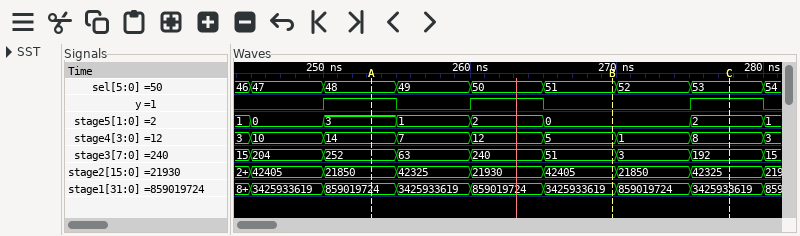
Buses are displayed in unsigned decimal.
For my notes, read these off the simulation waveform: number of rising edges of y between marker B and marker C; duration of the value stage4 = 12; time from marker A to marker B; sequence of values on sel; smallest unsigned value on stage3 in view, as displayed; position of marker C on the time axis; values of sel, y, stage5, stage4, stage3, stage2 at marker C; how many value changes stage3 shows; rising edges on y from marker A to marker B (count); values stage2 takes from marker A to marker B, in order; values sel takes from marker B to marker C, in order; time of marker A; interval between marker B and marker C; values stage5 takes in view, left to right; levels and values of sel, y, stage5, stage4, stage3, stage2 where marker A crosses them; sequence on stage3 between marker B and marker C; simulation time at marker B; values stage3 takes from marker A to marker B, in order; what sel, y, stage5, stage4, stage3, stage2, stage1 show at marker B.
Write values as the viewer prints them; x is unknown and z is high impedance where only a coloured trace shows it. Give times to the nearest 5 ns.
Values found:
1
5 ns
15 ns
46, 47, 48, 49, 50, 51, 52, 53, 54
3
280 ns
sel=53, y=1, stage5=2, stage4=8, stage3=192, stage2=42325
8
1
21850, 42325, 21930, 42405
51, 52, 53
255 ns
10 ns
1, 0, 3, 1, 2, 0, 2, 1
sel=48, y=1, stage5=3, stage4=14, stage3=252, stage2=21850
51, 3, 192
270 ns
252, 63, 240, 51
sel=51, y=0, stage5=0, stage4=5, stage3=51, stage2=42405, stage1=3425933619
